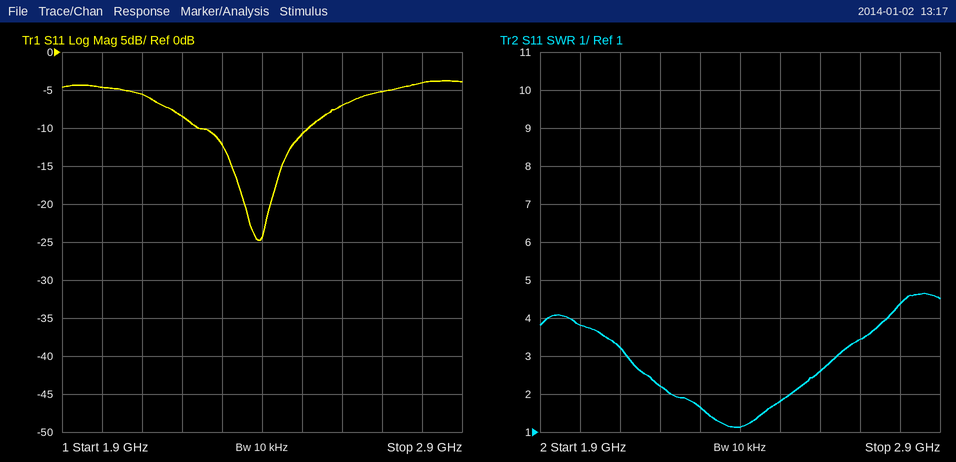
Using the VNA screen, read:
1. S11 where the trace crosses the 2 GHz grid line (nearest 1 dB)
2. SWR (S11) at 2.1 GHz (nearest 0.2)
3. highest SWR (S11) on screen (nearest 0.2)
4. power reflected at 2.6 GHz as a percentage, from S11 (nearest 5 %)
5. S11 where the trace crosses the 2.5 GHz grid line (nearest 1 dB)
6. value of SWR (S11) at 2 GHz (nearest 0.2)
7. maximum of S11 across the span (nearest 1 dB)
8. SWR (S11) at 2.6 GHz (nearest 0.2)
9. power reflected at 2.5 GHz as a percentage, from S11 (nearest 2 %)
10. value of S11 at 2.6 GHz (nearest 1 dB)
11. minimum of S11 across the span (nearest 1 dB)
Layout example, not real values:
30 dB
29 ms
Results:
-5 dB
3.2
4.6
20 %
-11 dB
3.8
-4 dB
2.6
8 %
-7 dB
-25 dB
